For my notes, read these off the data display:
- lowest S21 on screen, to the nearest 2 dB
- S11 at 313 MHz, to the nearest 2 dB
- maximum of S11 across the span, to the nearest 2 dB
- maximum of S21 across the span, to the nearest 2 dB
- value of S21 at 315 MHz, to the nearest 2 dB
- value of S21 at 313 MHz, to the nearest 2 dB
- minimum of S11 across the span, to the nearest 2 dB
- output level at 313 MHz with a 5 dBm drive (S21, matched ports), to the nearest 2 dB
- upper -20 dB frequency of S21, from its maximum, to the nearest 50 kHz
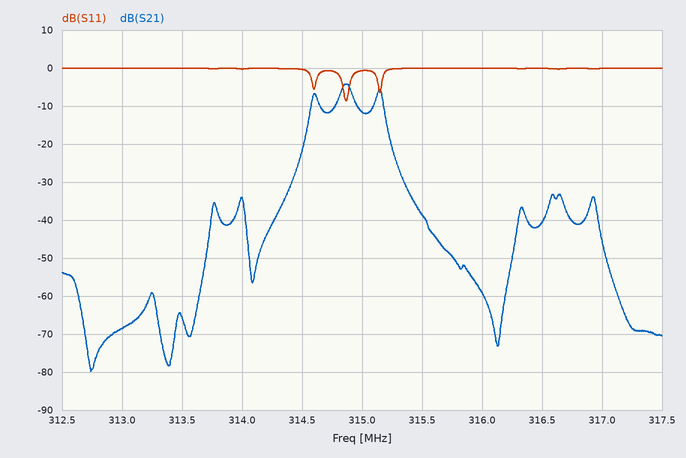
-80 dB
0 dB
0 dB
-4 dB
-12 dB
-68 dB
-8 dB
-64 dBm
315.30 MHz
